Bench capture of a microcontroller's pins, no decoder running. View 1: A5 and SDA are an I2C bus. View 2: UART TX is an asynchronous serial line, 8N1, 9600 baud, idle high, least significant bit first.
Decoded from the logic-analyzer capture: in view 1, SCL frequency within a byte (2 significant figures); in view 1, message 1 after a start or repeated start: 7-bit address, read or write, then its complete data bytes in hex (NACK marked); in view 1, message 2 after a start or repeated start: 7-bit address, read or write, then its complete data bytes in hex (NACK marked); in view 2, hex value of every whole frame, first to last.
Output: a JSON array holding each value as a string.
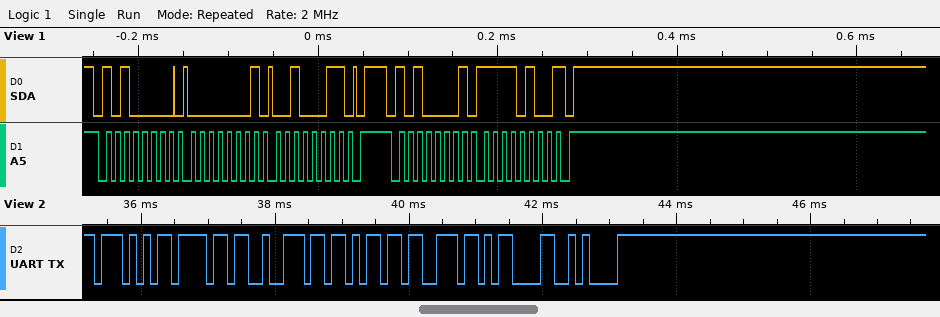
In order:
["100 kHz", "0x50 write: 01 23", "0x50 read: F4 NACK", "57 6F 72 6B 73 0D 0A"]
